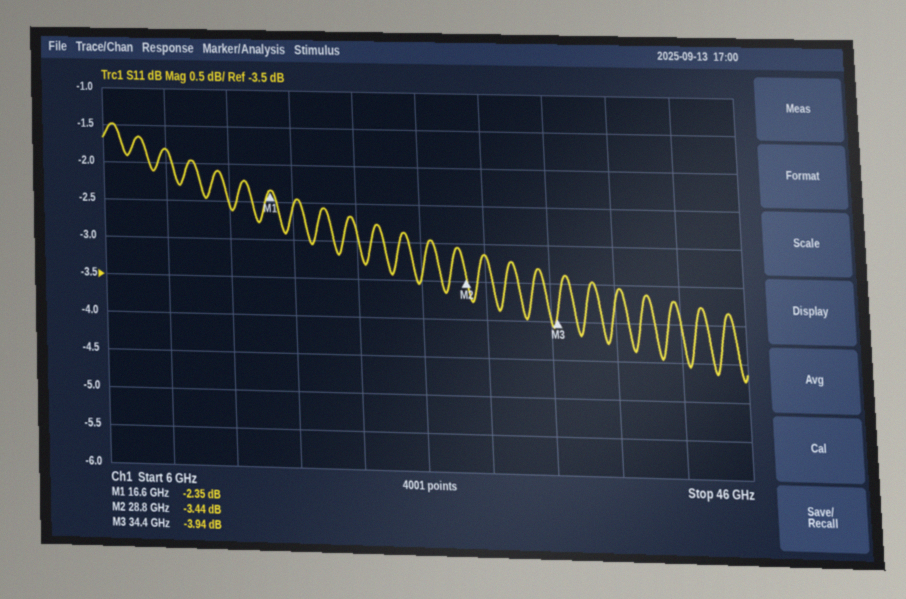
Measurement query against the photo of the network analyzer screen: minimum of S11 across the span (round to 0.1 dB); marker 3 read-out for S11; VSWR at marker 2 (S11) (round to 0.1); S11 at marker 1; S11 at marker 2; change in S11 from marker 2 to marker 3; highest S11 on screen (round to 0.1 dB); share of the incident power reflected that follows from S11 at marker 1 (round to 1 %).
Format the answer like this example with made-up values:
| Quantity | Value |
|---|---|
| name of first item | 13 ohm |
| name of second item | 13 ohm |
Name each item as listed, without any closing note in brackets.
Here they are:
| Quantity | Value |
|---|---|
| minimum of S11 across the span | -4.7 dB |
| marker 3 read-out for S11 | -3.94 dB |
| VSWR at marker 2 (S11) | 5.1 |
| S11 at marker 1 | -2.35 dB |
| S11 at marker 2 | -3.44 dB |
| change in S11 from marker 2 to marker 3 | -0.50 dB |
| highest S11 on screen | -1.5 dB |
| share of the incident power reflected that follows from S11 at marker 1 | 58 % |
